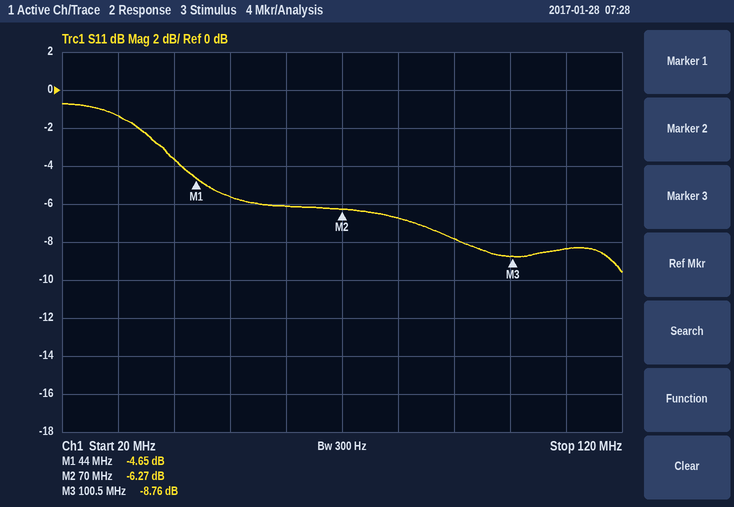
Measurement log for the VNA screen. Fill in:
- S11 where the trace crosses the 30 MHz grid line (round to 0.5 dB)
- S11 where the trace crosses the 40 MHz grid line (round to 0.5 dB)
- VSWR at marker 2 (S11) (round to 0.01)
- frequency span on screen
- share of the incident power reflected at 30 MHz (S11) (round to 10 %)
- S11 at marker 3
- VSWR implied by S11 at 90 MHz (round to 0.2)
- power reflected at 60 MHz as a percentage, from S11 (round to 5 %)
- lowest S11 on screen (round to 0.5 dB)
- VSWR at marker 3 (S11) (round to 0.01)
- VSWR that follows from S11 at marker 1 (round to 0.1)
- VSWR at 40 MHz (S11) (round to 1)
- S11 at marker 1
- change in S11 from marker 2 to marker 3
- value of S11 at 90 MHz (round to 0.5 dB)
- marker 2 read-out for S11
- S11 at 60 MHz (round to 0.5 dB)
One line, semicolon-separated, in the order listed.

-1.5 dB; -3.5 dB; 2.89; 100 MHz; 70 %; -8.76 dB; 2.4; 25 %; -9.5 dB; 2.15; 3.8; 5; -4.65 dB; -2.49 dB; -8.0 dB; -6.27 dB; -6.0 dB
